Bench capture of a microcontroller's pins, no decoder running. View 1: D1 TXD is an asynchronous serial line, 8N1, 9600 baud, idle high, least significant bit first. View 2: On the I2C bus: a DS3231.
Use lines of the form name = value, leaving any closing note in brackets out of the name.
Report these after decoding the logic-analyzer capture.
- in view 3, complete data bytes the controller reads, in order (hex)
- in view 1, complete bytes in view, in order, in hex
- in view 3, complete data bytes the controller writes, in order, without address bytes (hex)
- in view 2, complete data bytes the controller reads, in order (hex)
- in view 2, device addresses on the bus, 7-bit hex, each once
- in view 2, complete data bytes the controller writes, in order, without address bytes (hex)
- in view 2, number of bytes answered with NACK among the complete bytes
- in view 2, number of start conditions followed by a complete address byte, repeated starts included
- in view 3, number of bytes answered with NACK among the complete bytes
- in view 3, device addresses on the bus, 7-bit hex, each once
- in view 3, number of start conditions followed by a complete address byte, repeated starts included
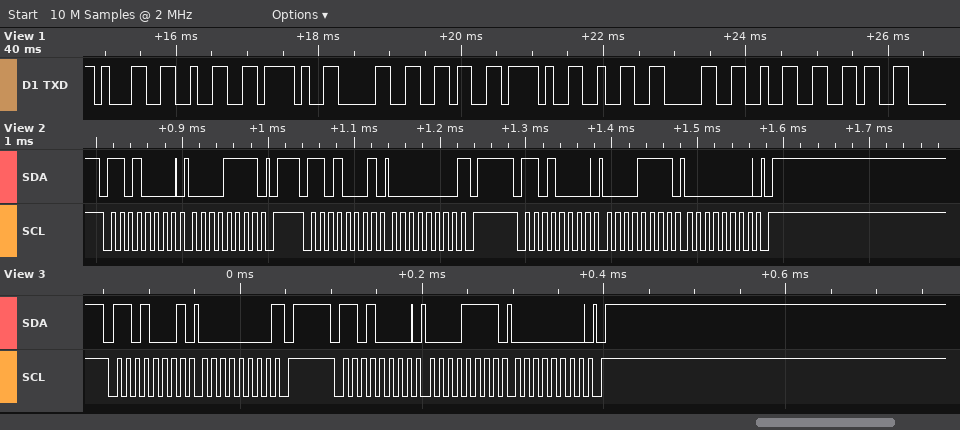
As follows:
in view 3, complete data bytes the controller reads, in order = 00
in view 1, complete bytes in view, in order, in hex = 31 32 2F 30 36 2F 32 30 32 36
in view 3, complete data bytes the controller writes, in order, without address bytes = 0F 00
in view 2, complete data bytes the controller reads, in order = 00
in view 2, device addresses on the bus, 7-bit hex, each once = 0x68
in view 2, complete data bytes the controller writes, in order, without address bytes = 0F 0F 00
in view 2, number of bytes answered with NACK among the complete bytes = 1
in view 2, number of start conditions followed by a complete address byte, repeated starts included = 3
in view 3, number of bytes answered with NACK among the complete bytes = 1
in view 3, device addresses on the bus, 7-bit hex, each once = 0x68
in view 3, number of start conditions followed by a complete address byte, repeated starts included = 2
